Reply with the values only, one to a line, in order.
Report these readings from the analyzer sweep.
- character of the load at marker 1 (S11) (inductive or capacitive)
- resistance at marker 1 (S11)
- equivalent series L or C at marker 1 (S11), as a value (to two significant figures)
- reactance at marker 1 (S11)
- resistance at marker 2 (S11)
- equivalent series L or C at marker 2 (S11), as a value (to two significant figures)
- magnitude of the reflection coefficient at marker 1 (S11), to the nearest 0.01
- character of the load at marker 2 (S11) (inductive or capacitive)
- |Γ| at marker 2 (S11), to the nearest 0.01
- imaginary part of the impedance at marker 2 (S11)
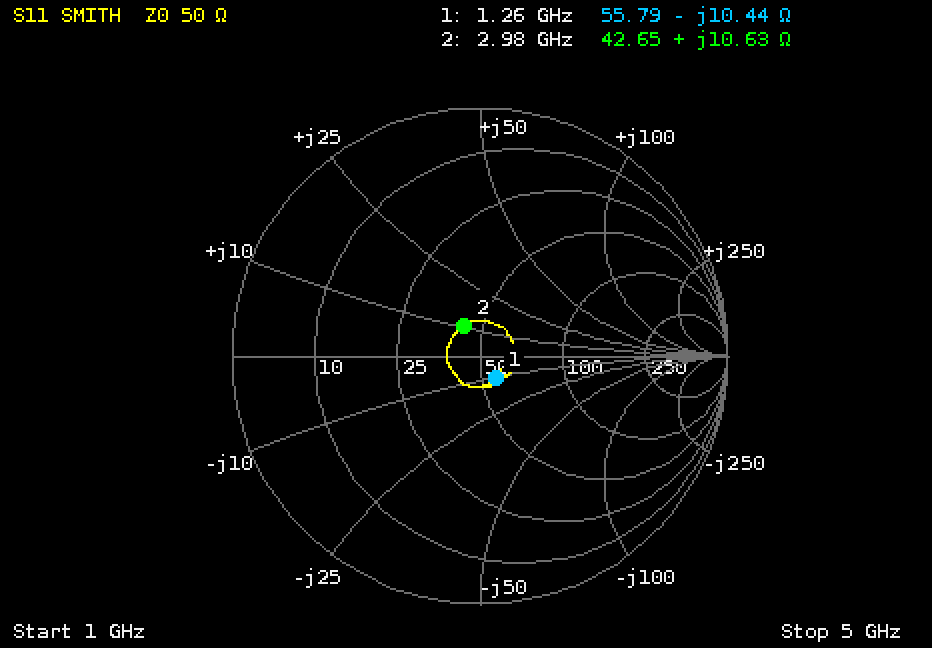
capacitive
55.79 Ω
12 pF
-10.44 Ω
42.65 Ω
570 pH
0.11
inductive
0.14
+10.63 Ω
